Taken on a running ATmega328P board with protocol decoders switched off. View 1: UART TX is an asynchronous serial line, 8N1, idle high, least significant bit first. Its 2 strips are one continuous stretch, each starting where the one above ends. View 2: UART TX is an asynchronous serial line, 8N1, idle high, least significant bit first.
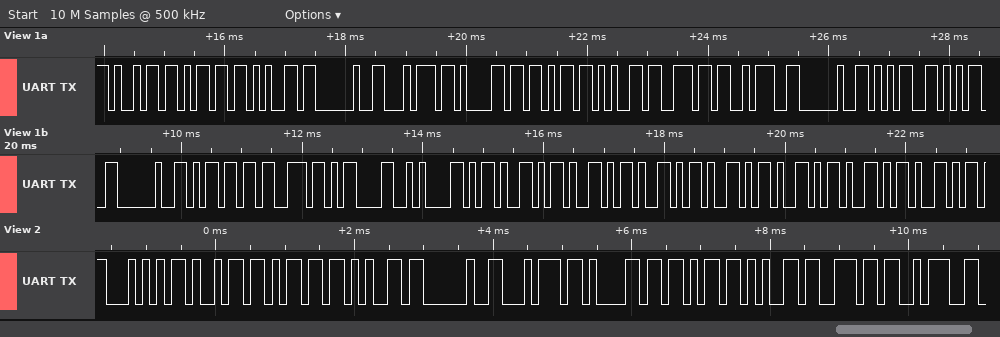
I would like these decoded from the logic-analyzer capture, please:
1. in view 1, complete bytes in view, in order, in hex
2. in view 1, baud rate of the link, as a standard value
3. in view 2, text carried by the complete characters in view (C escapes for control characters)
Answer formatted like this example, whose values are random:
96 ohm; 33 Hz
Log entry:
69 6D 65 20 74 61 6B 65 6E 3A 20 35 35 20 6D 73 0D 0A 2D 2D 2D 2D 2D 2D 2D; 9600 baud; "Time taken:"
